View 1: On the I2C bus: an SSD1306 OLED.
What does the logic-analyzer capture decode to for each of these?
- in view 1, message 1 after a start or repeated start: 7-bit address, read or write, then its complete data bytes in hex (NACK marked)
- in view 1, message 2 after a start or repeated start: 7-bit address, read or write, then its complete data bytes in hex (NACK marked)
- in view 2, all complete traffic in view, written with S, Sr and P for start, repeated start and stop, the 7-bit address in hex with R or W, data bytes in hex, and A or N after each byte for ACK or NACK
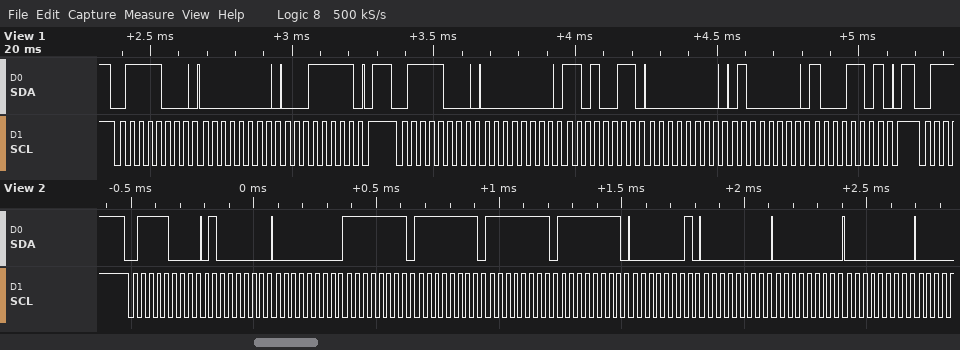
0x3C write: 00 1F
0x3C write: 00 D3 00 40 8D
S 3CW A 40 A 00 A FF A FF A FF A FF A 01 A 00 A 00 A 00 A
